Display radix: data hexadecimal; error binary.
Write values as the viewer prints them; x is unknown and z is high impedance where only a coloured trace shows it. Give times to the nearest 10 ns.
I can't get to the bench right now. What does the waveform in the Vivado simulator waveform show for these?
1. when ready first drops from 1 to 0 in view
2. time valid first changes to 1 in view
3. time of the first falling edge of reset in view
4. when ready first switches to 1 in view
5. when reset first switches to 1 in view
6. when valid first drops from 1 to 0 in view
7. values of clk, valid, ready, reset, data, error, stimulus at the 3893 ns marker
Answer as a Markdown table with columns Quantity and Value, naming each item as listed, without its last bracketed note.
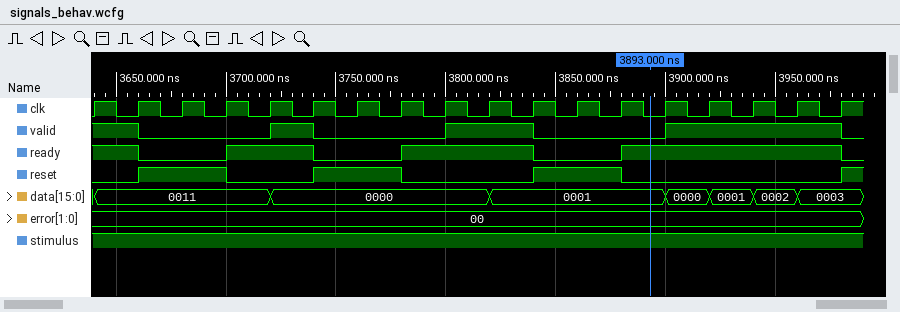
| Quantity | Value |
|---|---|
| when ready first drops from 1 to 0 in view | 3660 ns |
| time valid first changes to 1 in view | 3720 ns |
| time of the first falling edge of reset in view | 3700 ns |
| when ready first switches to 1 in view | 3700 ns |
| when reset first switches to 1 in view | 3660 ns |
| when valid first drops from 1 to 0 in view | 3660 ns |
| values of clk, valid, ready, reset, data, error, stimulus at the 3893 ns marker | clk=0, valid=0, ready=1, reset=0, data=0001, error=00, stimulus=1 |
